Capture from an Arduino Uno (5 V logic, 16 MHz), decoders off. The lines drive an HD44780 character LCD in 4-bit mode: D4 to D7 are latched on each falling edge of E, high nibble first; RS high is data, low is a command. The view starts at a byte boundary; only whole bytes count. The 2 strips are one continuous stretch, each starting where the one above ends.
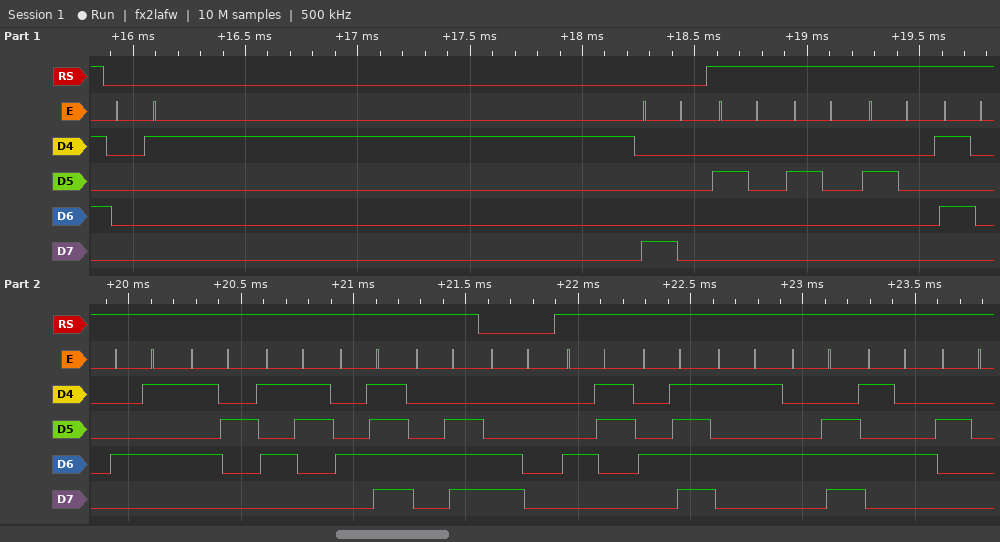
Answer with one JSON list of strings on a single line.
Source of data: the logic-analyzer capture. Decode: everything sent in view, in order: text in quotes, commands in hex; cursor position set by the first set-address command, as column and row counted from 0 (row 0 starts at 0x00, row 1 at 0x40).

["0x01 0x80 \"   PERSON\" 0xC0 \"COUNT \"", "column 0, row 0"]
